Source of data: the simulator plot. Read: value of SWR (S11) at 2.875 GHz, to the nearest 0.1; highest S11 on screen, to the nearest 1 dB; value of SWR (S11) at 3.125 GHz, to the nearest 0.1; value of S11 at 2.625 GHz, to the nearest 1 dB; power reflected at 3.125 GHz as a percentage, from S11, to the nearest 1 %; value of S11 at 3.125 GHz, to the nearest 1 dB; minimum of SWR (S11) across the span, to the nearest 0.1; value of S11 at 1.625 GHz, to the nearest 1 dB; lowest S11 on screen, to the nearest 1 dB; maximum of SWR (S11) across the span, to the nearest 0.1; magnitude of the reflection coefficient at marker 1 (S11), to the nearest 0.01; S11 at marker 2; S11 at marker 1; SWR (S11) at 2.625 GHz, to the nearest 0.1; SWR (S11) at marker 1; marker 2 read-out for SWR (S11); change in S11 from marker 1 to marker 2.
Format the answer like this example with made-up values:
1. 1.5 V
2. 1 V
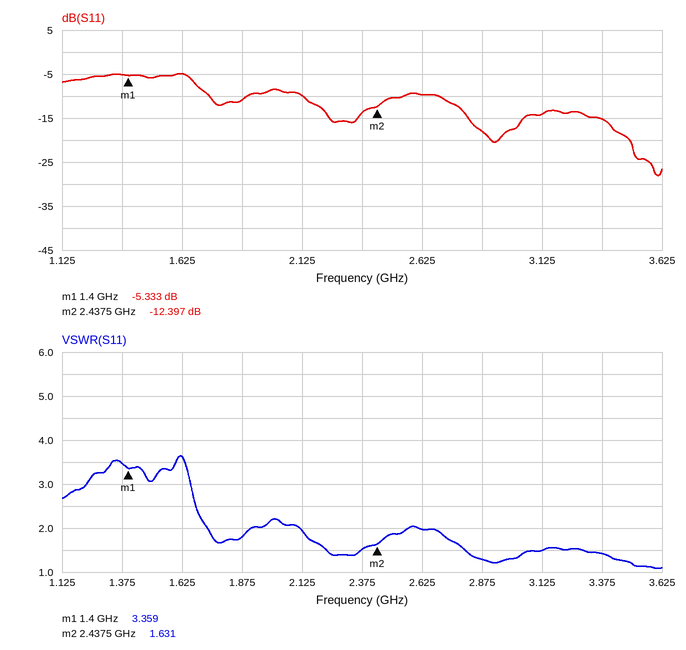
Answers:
1. 1.3
2. -5 dB
3. 1.5
4. -10 dB
5. 4 %
6. -14 dB
7. 1.1
8. -5 dB
9. -28 dB
10. 3.6
11. 0.54
12. -12.397 dB
13. -5.333 dB
14. 2.0
15. 3.359
16. 1.631
17. -7.064 dB
